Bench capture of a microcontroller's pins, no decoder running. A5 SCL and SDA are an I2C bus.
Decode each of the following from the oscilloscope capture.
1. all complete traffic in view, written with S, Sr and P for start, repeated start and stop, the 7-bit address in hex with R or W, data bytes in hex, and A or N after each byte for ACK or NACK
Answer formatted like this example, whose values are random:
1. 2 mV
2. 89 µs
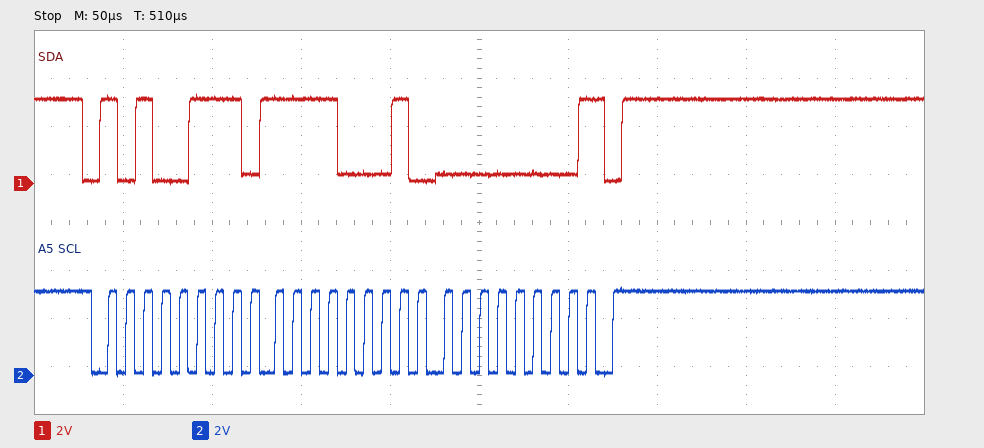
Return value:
1. S 53R A F1 A 00 N P
